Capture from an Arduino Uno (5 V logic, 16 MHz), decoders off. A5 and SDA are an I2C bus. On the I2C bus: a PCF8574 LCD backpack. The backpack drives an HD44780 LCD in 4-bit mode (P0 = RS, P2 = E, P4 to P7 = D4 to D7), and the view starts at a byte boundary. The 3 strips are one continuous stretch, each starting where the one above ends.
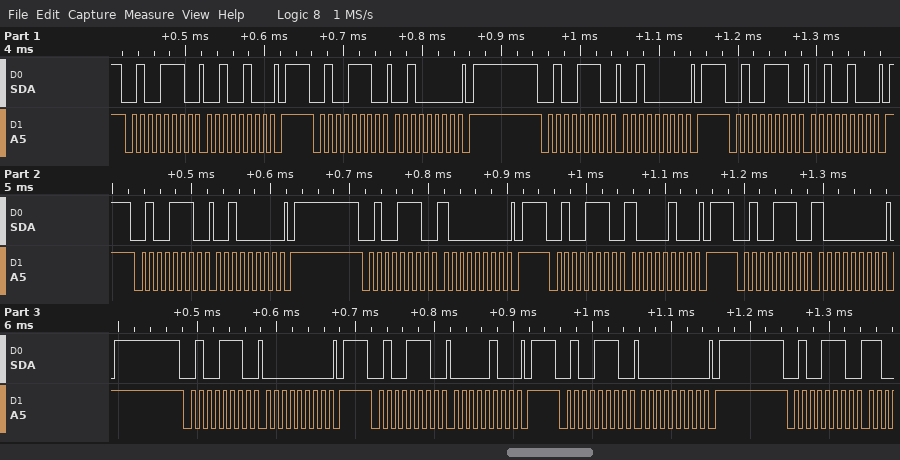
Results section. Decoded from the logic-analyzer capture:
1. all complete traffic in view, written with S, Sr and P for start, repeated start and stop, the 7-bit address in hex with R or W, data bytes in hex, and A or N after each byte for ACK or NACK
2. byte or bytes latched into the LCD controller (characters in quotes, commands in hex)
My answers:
S 27W A 24 A P S 27W A 20 A P S 27W A 20 A P S 27W A 24 A P S 27W A 20 A P S 27W A 80 A P S 27W A 84 A P S 27W A 80 A P S 27W A 00 A P S 27W A 04 A P S 27W A 00 A P S 27W A
0x28
